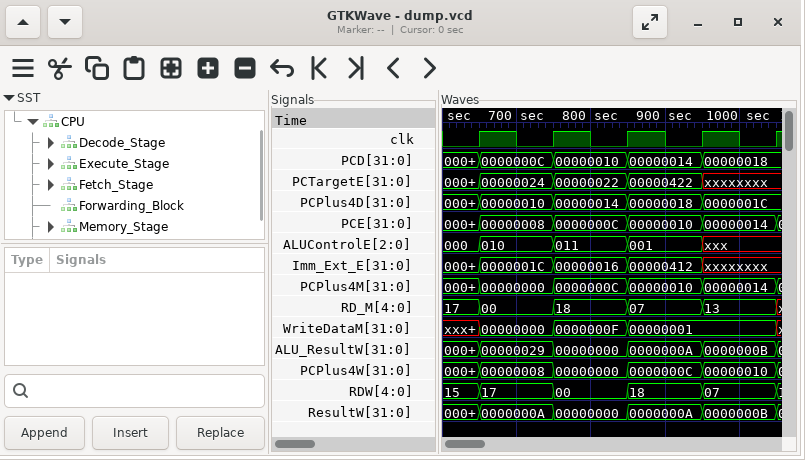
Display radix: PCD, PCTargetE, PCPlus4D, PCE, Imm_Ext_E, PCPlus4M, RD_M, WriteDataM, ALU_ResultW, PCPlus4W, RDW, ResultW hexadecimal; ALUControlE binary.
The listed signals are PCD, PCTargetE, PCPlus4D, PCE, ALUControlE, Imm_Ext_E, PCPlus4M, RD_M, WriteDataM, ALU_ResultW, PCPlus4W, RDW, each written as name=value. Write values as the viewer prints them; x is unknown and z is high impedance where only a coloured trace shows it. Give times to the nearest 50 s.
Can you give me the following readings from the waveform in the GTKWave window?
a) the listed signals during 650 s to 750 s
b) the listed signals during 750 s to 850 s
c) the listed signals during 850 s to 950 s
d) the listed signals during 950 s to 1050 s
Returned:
PCD=0000000C, PCTargetE=00000024, PCPlus4D=00000010, PCE=00000008, ALUControlE=010, Imm_Ext_E=0000001C, PCPlus4M=00000000, RD_M=00, WriteDataM=00000000, ALU_ResultW=00000029, PCPlus4W=00000008, RDW=17
PCD=00000010, PCTargetE=00000022, PCPlus4D=00000014, PCE=0000000C, ALUControlE=011, Imm_Ext_E=00000016, PCPlus4M=0000000C, RD_M=18, WriteDataM=0000000F, ALU_ResultW=00000000, PCPlus4W=00000000, RDW=00
PCD=00000014, PCTargetE=00000422, PCPlus4D=00000018, PCE=00000010, ALUControlE=001, Imm_Ext_E=00000412, PCPlus4M=00000010, RD_M=07, WriteDataM=00000001, ALU_ResultW=0000000A, PCPlus4W=0000000C, RDW=18
PCD=00000018, PCTargetE=xxxxxxxx, PCPlus4D=0000001C, PCE=00000014, ALUControlE=xxx, Imm_Ext_E=xxxxxxxx, PCPlus4M=00000014, RD_M=13, WriteDataM=00000001, ALU_ResultW=0000000B, PCPlus4W=00000010, RDW=07
